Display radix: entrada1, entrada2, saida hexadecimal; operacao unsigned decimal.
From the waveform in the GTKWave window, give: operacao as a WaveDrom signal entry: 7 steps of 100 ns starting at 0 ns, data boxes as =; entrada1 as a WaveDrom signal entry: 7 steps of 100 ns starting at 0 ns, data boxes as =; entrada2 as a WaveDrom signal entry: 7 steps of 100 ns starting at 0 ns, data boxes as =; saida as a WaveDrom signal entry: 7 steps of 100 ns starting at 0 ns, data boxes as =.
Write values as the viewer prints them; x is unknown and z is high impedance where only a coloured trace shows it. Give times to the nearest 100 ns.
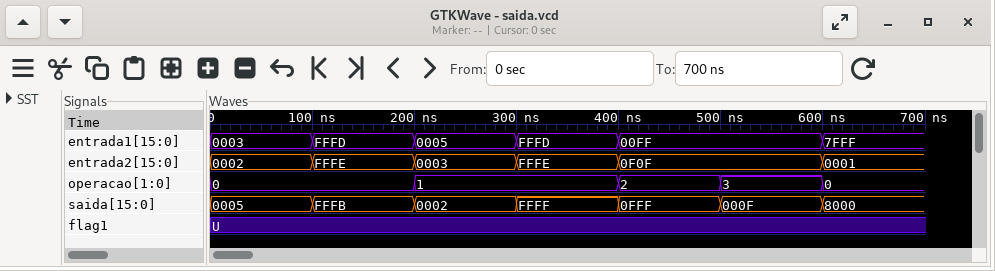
{name: 'operacao', wave: '=.=.===', data: '0 1 2 3 0'}
{name: 'entrada1', wave: '=====.=', data: '0003 FFFD 0005 FFFD 00FF 7FFF'}
{name: 'entrada2', wave: '=====.=', data: '0002 FFFE 0003 FFFE 0F0F 0001'}
{name: 'saida', wave: '=======', data: '0005 FFFB 0002 FFFF 0FFF 000F 8000'}
